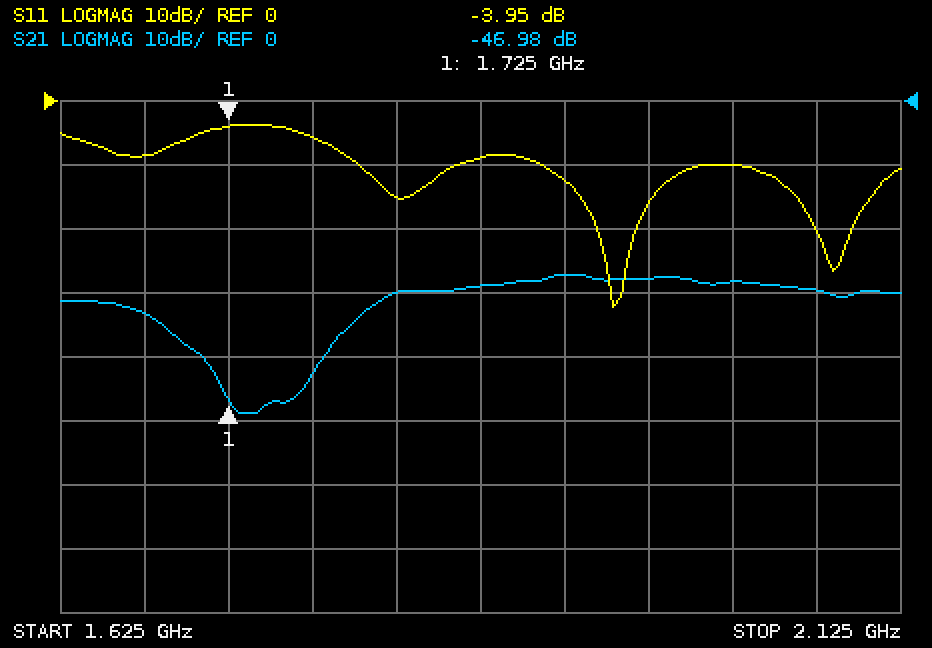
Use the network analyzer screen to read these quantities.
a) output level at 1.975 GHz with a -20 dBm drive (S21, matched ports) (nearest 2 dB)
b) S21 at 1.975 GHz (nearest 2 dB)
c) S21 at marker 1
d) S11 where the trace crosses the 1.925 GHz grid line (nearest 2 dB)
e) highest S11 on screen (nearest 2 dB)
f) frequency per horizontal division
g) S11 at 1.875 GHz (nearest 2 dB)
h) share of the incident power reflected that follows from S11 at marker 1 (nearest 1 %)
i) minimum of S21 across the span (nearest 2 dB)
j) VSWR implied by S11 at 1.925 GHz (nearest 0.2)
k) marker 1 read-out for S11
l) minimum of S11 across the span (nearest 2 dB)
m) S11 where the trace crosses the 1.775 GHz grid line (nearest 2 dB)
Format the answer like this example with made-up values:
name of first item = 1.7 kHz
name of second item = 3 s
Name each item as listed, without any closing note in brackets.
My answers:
output level at 1.975 GHz with a -20 dBm drive (S21, matched ports) = -48 dBm
S21 at 1.975 GHz = -28 dB
S21 at marker 1 = -46.98 dB
S11 where the trace crosses the 1.925 GHz grid line = -12 dB
highest S11 on screen = -4 dB
frequency per horizontal division = 50 MHz
S11 at 1.875 GHz = -8 dB
share of the incident power reflected that follows from S11 at marker 1 = 40 %
minimum of S21 across the span = -48 dB
VSWR implied by S11 at 1.925 GHz = 1.6
marker 1 read-out for S11 = -3.95 dB
minimum of S11 across the span = -32 dB
S11 where the trace crosses the 1.775 GHz grid line = -6 dB
